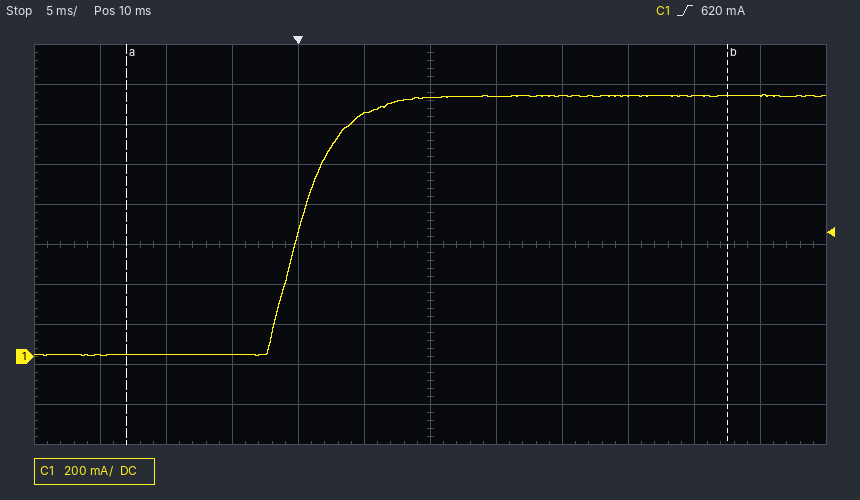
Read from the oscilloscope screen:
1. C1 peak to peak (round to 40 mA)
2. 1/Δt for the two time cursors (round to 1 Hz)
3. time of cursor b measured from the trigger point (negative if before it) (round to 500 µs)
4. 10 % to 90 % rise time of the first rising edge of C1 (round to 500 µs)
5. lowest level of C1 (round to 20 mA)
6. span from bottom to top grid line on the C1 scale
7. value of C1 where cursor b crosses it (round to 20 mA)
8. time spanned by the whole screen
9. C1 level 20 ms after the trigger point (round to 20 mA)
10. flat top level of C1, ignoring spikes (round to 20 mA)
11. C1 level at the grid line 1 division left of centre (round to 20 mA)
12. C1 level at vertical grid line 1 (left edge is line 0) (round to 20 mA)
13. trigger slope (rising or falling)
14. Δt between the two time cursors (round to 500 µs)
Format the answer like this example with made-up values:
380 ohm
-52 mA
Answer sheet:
1.32 A
22 Hz
+32.5 ms
6.0 ms
0 mA
2 A
1.30 A
60 ms
1.30 A
1.30 A
1.22 A
0 mA
rising
45.5 ms
